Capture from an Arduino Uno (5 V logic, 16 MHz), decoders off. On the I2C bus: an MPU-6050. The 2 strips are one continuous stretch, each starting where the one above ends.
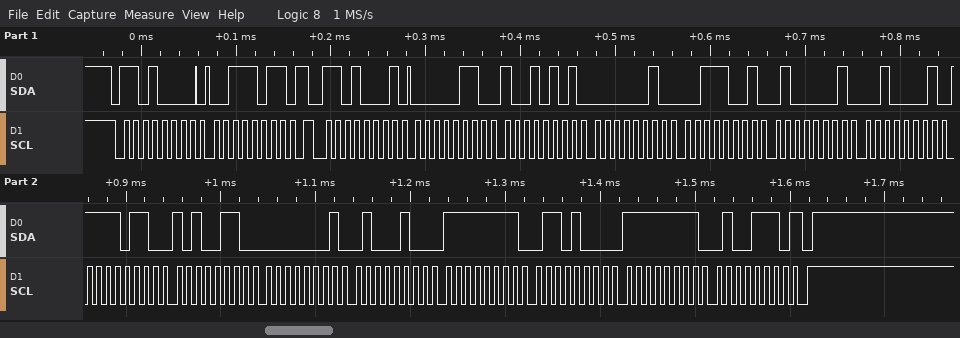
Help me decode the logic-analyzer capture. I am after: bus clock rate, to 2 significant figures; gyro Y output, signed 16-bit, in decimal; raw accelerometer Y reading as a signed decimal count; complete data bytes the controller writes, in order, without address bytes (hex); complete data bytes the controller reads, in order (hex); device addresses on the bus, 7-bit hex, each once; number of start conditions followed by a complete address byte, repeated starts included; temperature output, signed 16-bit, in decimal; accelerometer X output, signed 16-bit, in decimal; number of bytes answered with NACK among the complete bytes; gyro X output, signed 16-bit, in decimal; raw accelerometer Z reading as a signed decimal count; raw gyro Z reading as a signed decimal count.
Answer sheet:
100 kHz
-152
569
3B
06 95 02 39 41 21 F6 A6 01 44 FF 68 FF 4E
0x68
2
-2394
1685
1
324
16673
-178
